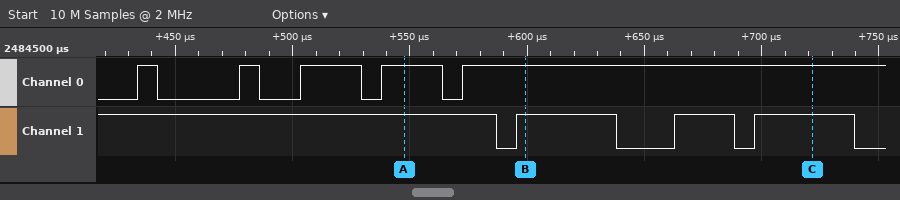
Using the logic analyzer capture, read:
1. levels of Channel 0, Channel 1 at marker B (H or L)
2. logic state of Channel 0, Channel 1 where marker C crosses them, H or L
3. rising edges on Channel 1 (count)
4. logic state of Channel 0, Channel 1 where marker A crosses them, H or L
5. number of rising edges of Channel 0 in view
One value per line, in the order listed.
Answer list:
Channel 0=H, Channel 1=H
Channel 0=H, Channel 1=H
3
Channel 0=H, Channel 1=H
5
